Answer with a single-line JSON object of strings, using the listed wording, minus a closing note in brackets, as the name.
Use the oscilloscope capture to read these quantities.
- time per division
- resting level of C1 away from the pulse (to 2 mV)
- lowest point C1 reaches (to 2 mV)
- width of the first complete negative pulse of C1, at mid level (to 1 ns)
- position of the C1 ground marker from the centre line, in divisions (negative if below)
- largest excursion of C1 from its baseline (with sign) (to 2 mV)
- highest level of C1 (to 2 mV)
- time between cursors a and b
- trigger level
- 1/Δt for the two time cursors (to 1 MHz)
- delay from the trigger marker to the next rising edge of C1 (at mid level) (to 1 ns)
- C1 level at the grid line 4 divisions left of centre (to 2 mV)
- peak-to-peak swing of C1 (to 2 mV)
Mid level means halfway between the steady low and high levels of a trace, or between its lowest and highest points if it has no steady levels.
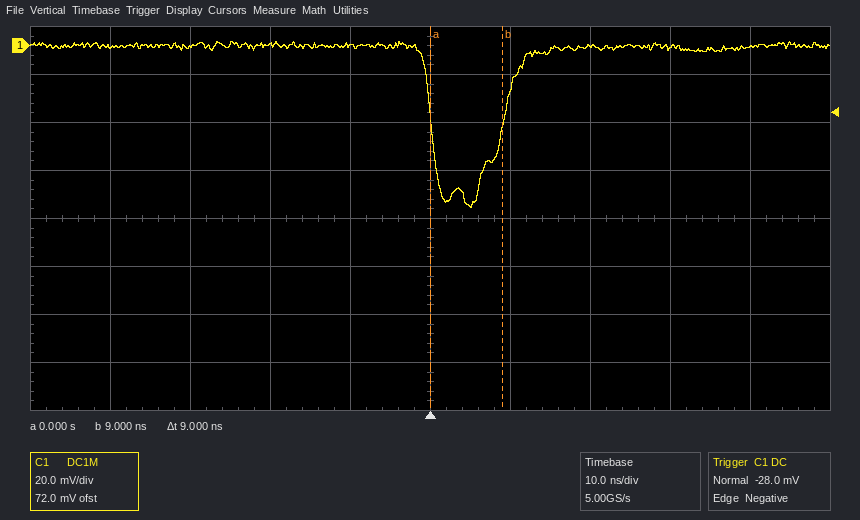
{"time per division": "10 ns", "resting level of C1 away from the pulse": "0 mV", "lowest point C1 reaches": "-68 mV", "width of the first complete negative pulse of C1, at mid level": "9 ns", "position of the C1 ground marker from the centre line, in divisions": "+3.6 div", "largest excursion of C1 from its baseline (with sign)": "-68 mV", "highest level of C1": "2 mV", "time between cursors a and b": "9 ns", "trigger level": "-28.0 mV", "1/Δt for the two time cursors": "111 MHz", "delay from the trigger marker to the next rising edge of C1 (at mid level)": "9 ns", "C1 level at the grid line 4 divisions left of centre": "0 mV", "peak-to-peak swing of C1": "70 mV"}
